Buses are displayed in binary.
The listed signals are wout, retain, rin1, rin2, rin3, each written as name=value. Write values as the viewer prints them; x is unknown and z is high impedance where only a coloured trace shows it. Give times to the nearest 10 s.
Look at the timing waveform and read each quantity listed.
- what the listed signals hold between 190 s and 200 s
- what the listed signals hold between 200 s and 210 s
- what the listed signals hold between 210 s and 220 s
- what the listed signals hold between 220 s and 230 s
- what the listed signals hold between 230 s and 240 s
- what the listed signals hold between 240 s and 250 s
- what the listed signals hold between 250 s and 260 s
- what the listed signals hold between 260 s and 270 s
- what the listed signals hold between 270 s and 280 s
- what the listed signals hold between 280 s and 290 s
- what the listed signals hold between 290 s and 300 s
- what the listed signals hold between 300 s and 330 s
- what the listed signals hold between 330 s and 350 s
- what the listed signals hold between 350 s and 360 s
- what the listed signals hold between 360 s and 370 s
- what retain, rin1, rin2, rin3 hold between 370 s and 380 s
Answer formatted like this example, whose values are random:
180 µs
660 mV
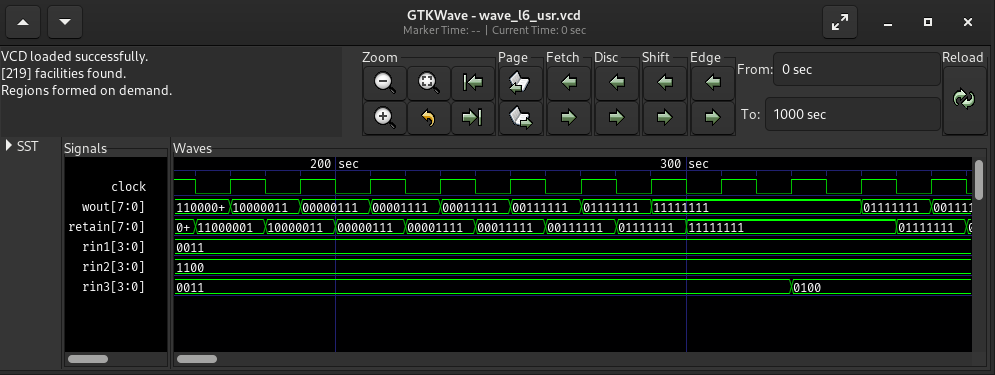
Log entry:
wout=00000111, retain=10000011, rin1=0011, rin2=1100, rin3=0011
wout=00000111, retain=00000111, rin1=0011, rin2=1100, rin3=0011
wout=00001111, retain=00000111, rin1=0011, rin2=1100, rin3=0011
wout=00001111, retain=00001111, rin1=0011, rin2=1100, rin3=0011
wout=00011111, retain=00001111, rin1=0011, rin2=1100, rin3=0011
wout=00011111, retain=00011111, rin1=0011, rin2=1100, rin3=0011
wout=00111111, retain=00011111, rin1=0011, rin2=1100, rin3=0011
wout=00111111, retain=00111111, rin1=0011, rin2=1100, rin3=0011
wout=01111111, retain=00111111, rin1=0011, rin2=1100, rin3=0011
wout=01111111, retain=01111111, rin1=0011, rin2=1100, rin3=0011
wout=11111111, retain=01111111, rin1=0011, rin2=1100, rin3=0011
wout=11111111, retain=11111111, rin1=0011, rin2=1100, rin3=0011
wout=11111111, retain=11111111, rin1=0011, rin2=1100, rin3=0100
wout=01111111, retain=11111111, rin1=0011, rin2=1100, rin3=0100
wout=01111111, retain=01111111, rin1=0011, rin2=1100, rin3=0100
retain=01111111, rin1=0011, rin2=1100, rin3=0100
